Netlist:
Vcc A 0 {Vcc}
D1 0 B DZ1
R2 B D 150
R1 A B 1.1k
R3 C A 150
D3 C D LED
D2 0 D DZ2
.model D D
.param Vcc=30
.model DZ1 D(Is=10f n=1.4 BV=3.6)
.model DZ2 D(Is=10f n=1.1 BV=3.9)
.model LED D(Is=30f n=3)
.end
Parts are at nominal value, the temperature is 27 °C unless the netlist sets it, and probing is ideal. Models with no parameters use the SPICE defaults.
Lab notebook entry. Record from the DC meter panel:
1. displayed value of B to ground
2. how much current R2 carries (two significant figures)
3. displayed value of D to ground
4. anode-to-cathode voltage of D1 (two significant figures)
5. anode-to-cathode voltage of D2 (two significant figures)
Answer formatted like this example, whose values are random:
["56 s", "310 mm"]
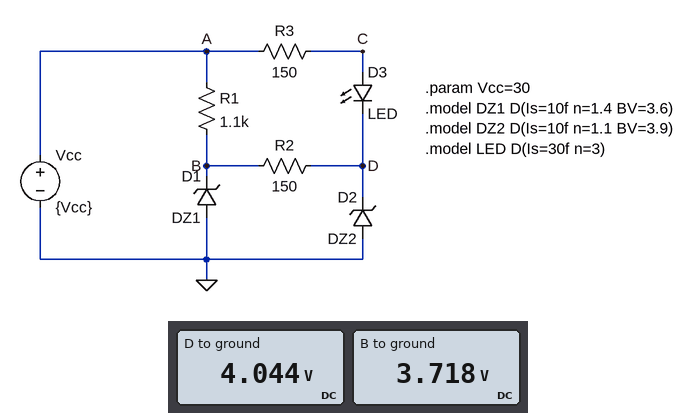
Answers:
["3.718 V", "2.2 mA", "4.044 V", "-3.7 V", "-4.0 V"]
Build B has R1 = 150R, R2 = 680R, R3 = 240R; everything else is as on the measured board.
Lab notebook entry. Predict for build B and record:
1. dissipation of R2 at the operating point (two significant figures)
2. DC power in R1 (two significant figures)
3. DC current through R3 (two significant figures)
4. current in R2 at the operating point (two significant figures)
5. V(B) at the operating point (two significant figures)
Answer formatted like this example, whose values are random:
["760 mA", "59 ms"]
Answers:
["87 µW", "4.6 W", "99 mA", "360 µA", "3.8 V"]
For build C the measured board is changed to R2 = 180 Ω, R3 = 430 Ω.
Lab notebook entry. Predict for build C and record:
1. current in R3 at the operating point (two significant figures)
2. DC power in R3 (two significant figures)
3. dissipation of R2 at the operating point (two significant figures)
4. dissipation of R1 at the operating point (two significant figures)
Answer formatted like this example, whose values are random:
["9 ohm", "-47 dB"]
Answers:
["55 mA", "1.3 W", "490 µW", "630 mW"]
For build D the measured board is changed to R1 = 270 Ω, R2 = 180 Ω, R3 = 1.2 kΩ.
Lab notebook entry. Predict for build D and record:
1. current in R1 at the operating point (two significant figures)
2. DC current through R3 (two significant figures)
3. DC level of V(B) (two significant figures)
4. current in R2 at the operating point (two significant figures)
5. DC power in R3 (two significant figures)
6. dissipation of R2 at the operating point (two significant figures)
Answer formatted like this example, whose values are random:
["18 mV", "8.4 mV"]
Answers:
["97 mA", "20 mA", "3.8 V", "1.2 mA", "480 mW", "260 µW"]
